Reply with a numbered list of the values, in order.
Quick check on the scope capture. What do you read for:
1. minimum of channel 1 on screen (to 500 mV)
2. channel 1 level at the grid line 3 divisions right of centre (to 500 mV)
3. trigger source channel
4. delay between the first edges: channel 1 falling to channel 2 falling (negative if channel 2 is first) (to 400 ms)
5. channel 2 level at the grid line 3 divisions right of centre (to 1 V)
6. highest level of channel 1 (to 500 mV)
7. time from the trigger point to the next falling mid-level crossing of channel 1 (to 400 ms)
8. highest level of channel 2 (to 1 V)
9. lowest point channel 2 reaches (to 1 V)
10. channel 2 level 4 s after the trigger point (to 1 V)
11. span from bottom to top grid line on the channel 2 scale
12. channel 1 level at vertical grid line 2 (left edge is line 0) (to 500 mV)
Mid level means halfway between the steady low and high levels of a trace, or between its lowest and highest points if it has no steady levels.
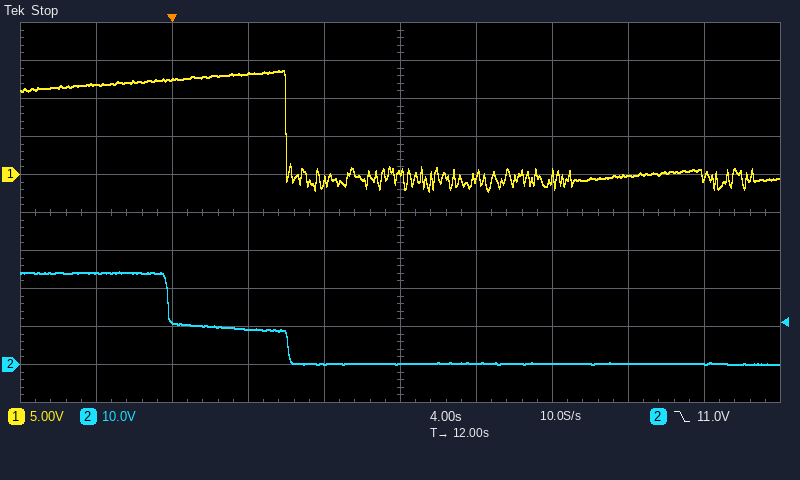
1. -2.0 V
2. 0.0 V
3. channel 2
4. -6.0 s
5. 0 V
6. 13.5 V
7. 6.0 s
8. 24 V
9. 0 V
10. 9 V
11. 100 V
12. 12.5 V
